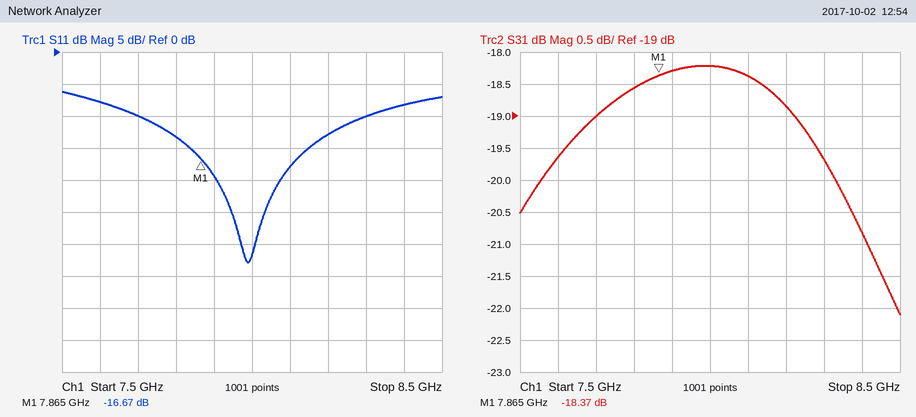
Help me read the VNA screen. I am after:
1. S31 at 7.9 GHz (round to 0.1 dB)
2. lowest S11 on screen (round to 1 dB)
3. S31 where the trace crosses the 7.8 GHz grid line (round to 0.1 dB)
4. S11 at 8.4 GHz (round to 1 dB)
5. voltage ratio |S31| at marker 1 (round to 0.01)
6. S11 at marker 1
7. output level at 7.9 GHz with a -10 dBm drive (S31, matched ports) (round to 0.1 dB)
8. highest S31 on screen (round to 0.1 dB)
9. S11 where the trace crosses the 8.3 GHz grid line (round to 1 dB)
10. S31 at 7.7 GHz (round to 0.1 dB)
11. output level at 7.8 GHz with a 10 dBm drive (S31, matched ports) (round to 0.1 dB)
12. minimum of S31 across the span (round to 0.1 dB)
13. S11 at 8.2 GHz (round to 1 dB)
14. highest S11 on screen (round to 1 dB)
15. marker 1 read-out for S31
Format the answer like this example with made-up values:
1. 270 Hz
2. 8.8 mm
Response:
1. -18.3 dB
2. -33 dB
3. -18.6 dB
4. -8 dB
5. 0.12
6. -16.67 dB
7. -28.3 dBm
8. -18.2 dB
9. -10 dB
10. -19.0 dB
11. -8.6 dBm
12. -22.1 dB
13. -13 dB
14. -6 dB
15. -18.37 dB
